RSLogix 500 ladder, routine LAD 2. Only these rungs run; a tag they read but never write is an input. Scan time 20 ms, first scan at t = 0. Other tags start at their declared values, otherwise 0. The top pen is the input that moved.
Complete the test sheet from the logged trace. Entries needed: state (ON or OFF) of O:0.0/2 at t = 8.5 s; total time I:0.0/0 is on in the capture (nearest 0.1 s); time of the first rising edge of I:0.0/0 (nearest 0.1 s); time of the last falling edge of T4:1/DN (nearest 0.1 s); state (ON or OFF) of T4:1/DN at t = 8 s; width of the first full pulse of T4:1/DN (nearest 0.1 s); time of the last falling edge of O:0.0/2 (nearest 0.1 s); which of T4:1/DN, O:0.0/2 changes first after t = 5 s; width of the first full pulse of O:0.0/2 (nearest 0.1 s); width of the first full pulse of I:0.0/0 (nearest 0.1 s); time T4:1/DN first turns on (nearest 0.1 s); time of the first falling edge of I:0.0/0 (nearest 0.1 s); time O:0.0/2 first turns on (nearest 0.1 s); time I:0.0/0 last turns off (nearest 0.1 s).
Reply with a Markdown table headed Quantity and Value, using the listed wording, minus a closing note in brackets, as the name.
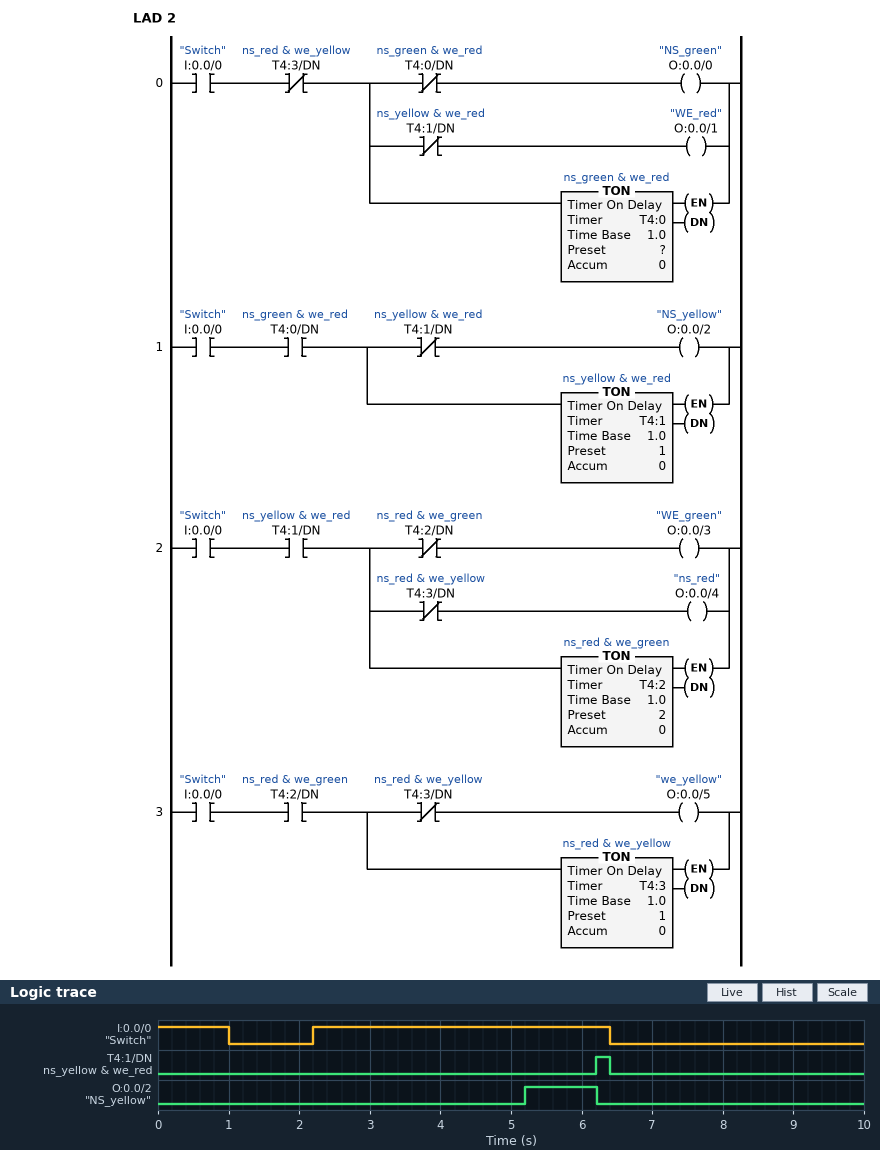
| Quantity | Value |
|---|---|
| state (ON or OFF) of O:0.0/2 at t = 8.5 s | OFF |
| total time I:0.0/0 is on in the capture | 5.2 s |
| time of the first rising edge of I:0.0/0 | 2.2 s |
| time of the last falling edge of T4:1/DN | 6.4 s |
| state (ON or OFF) of T4:1/DN at t = 8 s | OFF |
| width of the first full pulse of T4:1/DN | 0.2 s |
| time of the last falling edge of O:0.0/2 | 6.2 s |
| which of T4:1/DN, O:0.0/2 changes first after t = 5 s | O:0.0/2 |
| width of the first full pulse of O:0.0/2 | 1.0 s |
| width of the first full pulse of I:0.0/0 | 4.2 s |
| time T4:1/DN first turns on | 6.2 s |
| time of the first falling edge of I:0.0/0 | 1.0 s |
| time O:0.0/2 first turns on | 5.2 s |
| time I:0.0/0 last turns off | 6.4 s |
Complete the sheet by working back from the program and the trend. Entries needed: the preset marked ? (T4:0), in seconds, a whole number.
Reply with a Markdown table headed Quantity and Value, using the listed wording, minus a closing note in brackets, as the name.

| Quantity | Value |
|---|---|
| the preset marked ? (T4:0), in seconds, a whole number | 3 s |
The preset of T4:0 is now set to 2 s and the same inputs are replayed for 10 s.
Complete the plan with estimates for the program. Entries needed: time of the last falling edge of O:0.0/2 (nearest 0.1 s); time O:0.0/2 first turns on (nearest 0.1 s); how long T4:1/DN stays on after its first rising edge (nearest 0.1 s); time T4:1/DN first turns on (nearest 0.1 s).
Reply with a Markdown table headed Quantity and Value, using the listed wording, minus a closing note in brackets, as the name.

| Quantity | Value |
|---|---|
| time of the last falling edge of O:0.0/2 | 5.2 s |
| time O:0.0/2 first turns on | 4.2 s |
| how long T4:1/DN stays on after its first rising edge | 1.2 s |
| time T4:1/DN first turns on | 5.2 s |
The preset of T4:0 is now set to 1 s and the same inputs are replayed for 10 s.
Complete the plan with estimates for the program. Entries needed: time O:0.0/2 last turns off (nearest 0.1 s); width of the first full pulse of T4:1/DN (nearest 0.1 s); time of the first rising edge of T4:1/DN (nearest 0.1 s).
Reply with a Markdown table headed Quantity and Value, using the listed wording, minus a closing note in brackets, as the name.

| Quantity | Value |
|---|---|
| time O:0.0/2 last turns off | 4.2 s |
| width of the first full pulse of T4:1/DN | 2.2 s |
| time of the first rising edge of T4:1/DN | 4.2 s |
